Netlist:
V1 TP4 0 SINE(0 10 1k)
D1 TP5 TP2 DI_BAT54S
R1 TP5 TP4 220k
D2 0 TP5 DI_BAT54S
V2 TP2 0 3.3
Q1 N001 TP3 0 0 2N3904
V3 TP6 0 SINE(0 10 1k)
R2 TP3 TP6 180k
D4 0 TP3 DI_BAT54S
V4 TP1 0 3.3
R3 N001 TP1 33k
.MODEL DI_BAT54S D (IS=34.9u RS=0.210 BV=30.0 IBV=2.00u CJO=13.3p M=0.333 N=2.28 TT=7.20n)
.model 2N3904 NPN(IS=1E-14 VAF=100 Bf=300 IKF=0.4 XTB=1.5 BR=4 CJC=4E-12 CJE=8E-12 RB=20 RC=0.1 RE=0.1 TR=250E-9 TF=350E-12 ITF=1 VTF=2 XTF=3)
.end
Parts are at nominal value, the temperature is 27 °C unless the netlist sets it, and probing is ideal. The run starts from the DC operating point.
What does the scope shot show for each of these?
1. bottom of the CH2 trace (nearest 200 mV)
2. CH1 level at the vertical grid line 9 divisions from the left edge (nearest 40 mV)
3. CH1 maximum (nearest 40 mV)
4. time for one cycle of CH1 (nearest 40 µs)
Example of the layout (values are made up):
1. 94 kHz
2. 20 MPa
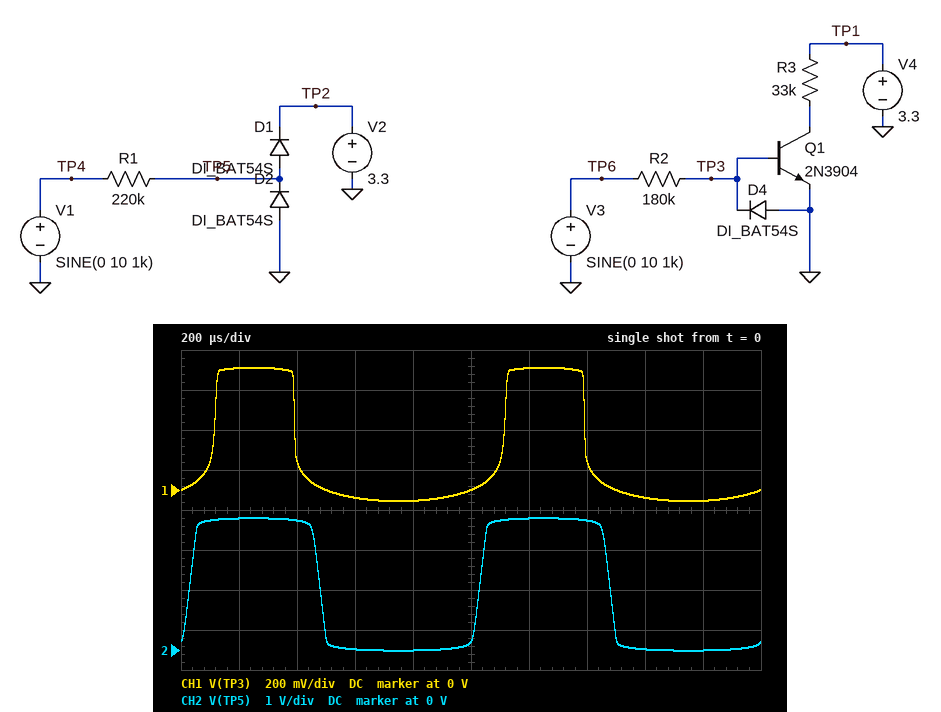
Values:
1. 0 V
2. -40 mV
3. 600 mV
4. 1.00 ms
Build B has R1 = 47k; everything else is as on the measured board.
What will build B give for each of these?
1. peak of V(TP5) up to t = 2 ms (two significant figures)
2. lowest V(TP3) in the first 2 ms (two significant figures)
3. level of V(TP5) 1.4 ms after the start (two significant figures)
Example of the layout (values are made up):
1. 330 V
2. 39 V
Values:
1. 3.4 V
2. -56 mV
3. 3.3 V
